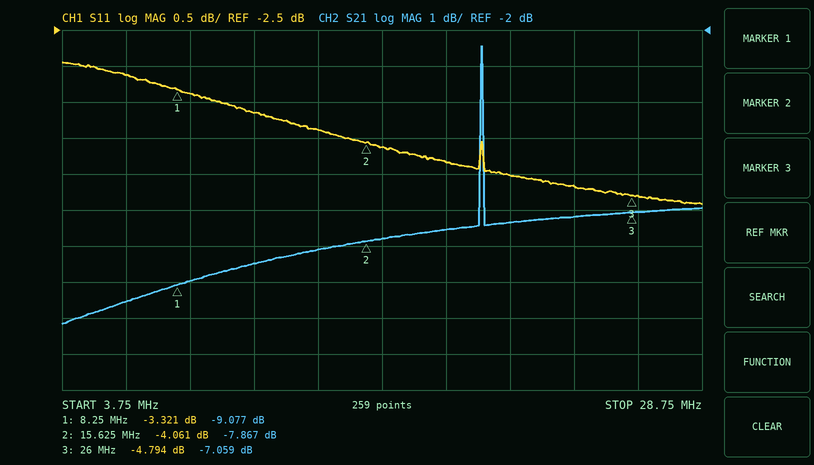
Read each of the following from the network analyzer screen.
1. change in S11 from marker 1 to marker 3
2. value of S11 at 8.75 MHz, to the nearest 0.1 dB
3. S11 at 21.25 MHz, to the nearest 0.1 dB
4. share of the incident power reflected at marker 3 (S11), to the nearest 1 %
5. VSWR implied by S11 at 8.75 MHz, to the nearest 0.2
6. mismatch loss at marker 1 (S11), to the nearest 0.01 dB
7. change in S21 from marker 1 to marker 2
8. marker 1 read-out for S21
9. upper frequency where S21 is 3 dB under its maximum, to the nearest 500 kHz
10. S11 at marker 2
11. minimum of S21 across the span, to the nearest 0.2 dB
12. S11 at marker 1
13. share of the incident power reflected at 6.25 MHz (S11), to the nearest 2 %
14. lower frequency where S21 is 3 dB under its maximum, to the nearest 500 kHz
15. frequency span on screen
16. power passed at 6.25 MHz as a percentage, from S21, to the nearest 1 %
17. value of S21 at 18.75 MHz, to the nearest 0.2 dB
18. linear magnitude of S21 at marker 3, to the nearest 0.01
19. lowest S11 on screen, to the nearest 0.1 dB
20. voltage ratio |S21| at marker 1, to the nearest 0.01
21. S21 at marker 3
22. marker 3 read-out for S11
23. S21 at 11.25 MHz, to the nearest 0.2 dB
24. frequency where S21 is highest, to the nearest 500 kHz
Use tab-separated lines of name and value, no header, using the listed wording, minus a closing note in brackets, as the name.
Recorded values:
change in S11 from marker 1 to marker 3	-1.473 dB
value of S11 at 8.75 MHz, to the nearest 0.1 dB	-3.4 dB
S11 at 21.25 MHz, to the nearest 0.1 dB	-4.5 dB
share of the incident power reflected at marker 3 (S11), to the nearest 1 %	33 %
VSWR implied by S11 at 8.75 MHz, to the nearest 0.2	5.2
mismatch loss at marker 1 (S11), to the nearest 0.01 dB	2.72 dB
change in S21 from marker 1 to marker 2	1.210 dB
marker 1 read-out for S21	-9.077 dB
upper frequency where S21 is 3 dB under its maximum, to the nearest 500 kHz	20.0 MHz
S11 at marker 2	-4.061 dB
minimum of S21 across the span, to the nearest 0.2 dB	-10.2 dB
S11 at marker 1	-3.321 dB
share of the incident power reflected at 6.25 MHz (S11), to the nearest 2 %	48 %
lower frequency where S21 is 3 dB under its maximum, to the nearest 500 kHz	20.0 MHz
frequency span on screen	25 MHz
power passed at 6.25 MHz as a percentage, from S21, to the nearest 1 %	11 %
value of S21 at 18.75 MHz, to the nearest 0.2 dB	-7.6 dB
linear magnitude of S21 at marker 3, to the nearest 0.01	0.44
lowest S11 on screen, to the nearest 0.1 dB	-4.9 dB
voltage ratio |S21| at marker 1, to the nearest 0.01	0.35
S21 at marker 3	-7.059 dB
marker 3 read-out for S11	-4.794 dB
S21 at 11.25 MHz, to the nearest 0.2 dB	-8.4 dB
frequency where S21 is highest, to the nearest 500 kHz	20.0 MHz
